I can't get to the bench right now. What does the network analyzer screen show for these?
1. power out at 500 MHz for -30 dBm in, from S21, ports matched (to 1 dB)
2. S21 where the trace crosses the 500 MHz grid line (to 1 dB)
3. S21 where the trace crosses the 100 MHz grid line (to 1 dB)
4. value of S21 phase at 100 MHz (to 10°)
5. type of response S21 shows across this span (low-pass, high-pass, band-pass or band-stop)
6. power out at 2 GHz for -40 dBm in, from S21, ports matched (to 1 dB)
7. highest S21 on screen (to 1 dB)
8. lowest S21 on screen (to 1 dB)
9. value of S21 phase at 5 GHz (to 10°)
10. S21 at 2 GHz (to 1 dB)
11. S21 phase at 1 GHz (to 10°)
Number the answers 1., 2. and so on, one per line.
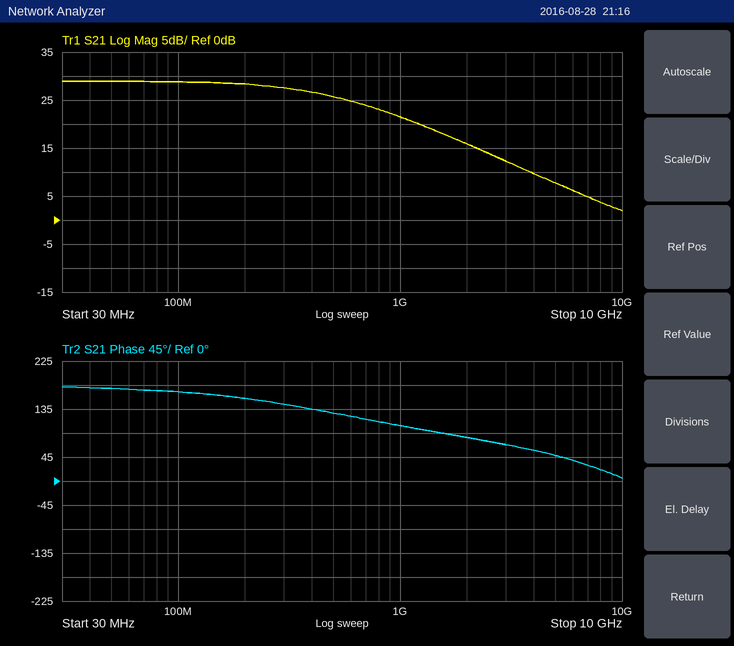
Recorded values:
1. -4 dBm
2. 26 dB
3. 29 dB
4. 170°
5. low-pass
6. -24 dBm
7. 29 dB
8. 2 dB
9. 50°
10. 16 dB
11. 100°
